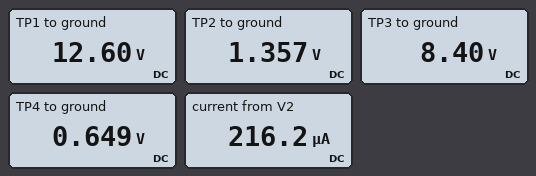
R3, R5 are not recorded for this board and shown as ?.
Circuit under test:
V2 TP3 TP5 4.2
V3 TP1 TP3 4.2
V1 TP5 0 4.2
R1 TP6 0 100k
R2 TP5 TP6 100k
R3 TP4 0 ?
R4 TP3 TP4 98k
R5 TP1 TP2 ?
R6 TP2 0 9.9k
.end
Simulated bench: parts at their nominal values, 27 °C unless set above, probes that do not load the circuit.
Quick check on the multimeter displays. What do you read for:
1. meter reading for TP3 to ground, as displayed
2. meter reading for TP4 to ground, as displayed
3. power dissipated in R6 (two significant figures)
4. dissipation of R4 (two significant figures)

8.40 V
0.649 V
190 µW
610 µW
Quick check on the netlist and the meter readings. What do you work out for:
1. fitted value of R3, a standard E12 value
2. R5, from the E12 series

8.2 kΩ
82 kΩ
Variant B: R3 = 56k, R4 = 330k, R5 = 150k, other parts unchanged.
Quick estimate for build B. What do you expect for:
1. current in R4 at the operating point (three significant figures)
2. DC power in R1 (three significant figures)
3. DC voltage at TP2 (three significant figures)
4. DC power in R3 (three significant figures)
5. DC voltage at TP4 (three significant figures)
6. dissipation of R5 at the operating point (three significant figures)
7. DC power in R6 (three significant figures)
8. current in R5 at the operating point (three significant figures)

21.8 µA
44.1 µW
780 mV
26.5 µW
1.22 V
931 µW
61.5 µW
78.8 µA
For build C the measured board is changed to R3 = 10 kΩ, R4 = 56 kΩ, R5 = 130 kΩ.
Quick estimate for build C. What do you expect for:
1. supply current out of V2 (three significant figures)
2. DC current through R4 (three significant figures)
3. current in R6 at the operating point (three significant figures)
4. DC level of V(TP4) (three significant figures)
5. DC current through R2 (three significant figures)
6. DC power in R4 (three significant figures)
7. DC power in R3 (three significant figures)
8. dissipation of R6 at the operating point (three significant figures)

217 µA
127 µA
90.1 µA
1.27 V
21.0 µA
907 µW
162 µW
80.3 µW
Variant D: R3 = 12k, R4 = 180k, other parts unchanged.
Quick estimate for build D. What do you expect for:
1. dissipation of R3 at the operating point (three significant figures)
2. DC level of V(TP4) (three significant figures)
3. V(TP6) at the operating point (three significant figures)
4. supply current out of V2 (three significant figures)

23.0 µW
525 mV
2.10 V
181 µA
